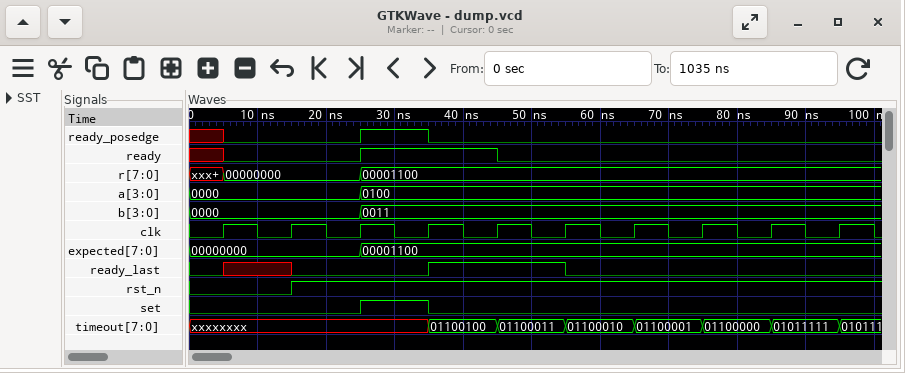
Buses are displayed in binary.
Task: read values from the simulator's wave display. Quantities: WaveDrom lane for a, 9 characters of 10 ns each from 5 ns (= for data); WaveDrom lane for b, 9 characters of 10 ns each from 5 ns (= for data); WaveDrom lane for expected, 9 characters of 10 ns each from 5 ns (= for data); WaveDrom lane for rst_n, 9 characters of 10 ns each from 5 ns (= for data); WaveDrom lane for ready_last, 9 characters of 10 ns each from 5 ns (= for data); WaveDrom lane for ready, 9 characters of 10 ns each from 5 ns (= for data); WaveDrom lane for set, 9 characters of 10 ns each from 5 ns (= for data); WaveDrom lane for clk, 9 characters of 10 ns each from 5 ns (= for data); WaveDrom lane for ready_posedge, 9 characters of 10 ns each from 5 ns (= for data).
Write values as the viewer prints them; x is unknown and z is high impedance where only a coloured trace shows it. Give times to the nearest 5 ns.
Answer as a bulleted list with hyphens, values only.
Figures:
- {name: 'a', wave: '=.=......', data: '0000 0100'}
- {name: 'b', wave: '=.=......', data: '0000 0011'}
- {name: 'expected', wave: '=.=......', data: '00000000 00001100'}
- {name: 'rst_n', wave: '01.......'}
- {name: 'ready_last', wave: 'x0.1.0...'}
- {name: 'ready', wave: '0.1.0....'}
- {name: 'set', wave: '0.10.....'}
- {name: 'clk', wave: 'p........'}
- {name: 'ready_posedge', wave: '0.10.....'}
